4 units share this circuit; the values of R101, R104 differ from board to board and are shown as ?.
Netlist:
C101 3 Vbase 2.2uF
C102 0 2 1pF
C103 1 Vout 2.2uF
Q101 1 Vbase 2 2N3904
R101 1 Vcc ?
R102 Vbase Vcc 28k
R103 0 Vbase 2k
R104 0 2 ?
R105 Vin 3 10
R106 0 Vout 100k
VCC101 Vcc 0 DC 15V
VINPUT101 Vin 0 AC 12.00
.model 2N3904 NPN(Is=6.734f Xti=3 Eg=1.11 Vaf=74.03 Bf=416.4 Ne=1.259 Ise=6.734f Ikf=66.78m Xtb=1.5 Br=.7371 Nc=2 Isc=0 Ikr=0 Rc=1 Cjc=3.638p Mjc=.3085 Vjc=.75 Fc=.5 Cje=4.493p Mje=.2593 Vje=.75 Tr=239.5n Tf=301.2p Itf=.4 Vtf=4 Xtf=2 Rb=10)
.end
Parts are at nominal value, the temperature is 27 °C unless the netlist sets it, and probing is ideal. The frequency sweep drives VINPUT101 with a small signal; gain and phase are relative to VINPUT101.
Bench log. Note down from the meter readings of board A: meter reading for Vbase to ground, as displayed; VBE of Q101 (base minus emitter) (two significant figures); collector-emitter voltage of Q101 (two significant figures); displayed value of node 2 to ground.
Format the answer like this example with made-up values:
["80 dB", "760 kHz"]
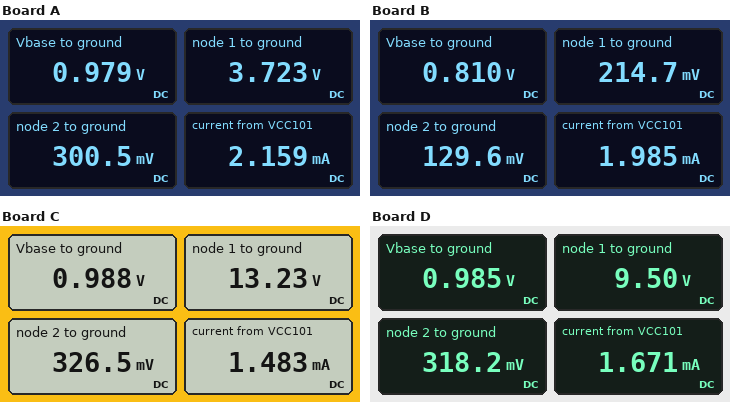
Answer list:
["0.979 V", "680 mV", "3.4 V", "300.5 mV"]
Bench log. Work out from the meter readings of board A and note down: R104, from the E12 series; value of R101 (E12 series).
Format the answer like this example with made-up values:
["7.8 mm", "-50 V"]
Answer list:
["180 Ω", "6.8 kΩ"]
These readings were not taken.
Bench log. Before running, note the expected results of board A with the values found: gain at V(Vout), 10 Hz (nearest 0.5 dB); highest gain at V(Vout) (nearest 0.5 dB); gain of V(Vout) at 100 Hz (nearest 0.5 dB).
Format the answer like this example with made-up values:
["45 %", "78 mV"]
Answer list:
["17.5 dB", "30.0 dB", "29.5 dB"]
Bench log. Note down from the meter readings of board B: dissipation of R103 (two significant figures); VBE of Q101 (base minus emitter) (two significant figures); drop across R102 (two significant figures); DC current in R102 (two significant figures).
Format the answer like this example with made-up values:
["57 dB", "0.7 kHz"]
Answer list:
["330 µW", "680 mV", "14 V", "510 µA"]
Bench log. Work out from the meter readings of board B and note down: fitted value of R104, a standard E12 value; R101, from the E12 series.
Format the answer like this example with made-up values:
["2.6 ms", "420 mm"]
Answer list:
["82 Ω", "10 kΩ"]
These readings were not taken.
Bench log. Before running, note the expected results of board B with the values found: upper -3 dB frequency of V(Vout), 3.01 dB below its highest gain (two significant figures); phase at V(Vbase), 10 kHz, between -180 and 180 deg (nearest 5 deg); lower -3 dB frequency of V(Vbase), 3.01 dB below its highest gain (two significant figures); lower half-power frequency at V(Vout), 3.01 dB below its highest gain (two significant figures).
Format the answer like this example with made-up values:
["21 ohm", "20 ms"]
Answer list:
["2.3 MHz", "5 deg", "580 Hz", "580 Hz"]
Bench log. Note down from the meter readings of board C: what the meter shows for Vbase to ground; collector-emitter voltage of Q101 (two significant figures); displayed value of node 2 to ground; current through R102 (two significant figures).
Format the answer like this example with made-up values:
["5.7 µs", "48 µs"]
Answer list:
["0.988 V", "13 V", "326.5 mV", "500 µA"]
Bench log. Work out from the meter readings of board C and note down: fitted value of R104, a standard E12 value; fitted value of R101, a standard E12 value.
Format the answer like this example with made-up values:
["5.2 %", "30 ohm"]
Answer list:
["330 Ω", "1.8 kΩ"]
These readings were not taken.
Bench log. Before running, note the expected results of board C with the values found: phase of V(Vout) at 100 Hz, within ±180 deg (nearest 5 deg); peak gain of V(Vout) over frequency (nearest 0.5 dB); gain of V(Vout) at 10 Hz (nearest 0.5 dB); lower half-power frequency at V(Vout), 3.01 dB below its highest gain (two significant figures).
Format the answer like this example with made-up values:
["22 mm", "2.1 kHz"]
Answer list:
["-160 deg", "14.0 dB", "1.5 dB", "40 Hz"]
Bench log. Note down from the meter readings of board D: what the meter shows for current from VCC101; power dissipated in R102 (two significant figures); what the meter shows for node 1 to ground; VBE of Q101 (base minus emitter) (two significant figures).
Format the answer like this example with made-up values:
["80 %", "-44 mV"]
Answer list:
["1.671 mA", "7.0 mW", "9.50 V", "670 mV"]
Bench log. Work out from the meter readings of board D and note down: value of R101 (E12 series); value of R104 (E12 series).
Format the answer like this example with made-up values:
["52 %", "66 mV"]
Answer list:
["4.7 kΩ", "270 Ω"]
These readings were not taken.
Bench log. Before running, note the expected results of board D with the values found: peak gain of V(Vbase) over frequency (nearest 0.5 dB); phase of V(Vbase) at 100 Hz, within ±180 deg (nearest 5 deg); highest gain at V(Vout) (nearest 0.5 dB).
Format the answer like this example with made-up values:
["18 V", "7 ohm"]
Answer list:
["0 dB", "20 deg", "23.5 dB"]
